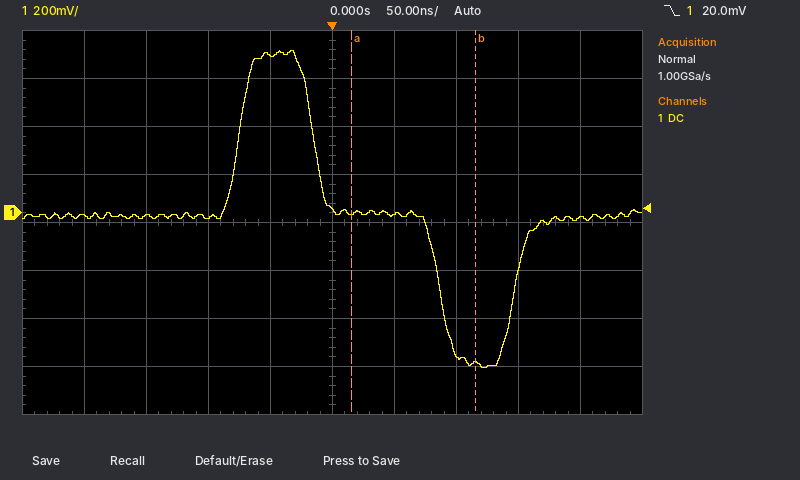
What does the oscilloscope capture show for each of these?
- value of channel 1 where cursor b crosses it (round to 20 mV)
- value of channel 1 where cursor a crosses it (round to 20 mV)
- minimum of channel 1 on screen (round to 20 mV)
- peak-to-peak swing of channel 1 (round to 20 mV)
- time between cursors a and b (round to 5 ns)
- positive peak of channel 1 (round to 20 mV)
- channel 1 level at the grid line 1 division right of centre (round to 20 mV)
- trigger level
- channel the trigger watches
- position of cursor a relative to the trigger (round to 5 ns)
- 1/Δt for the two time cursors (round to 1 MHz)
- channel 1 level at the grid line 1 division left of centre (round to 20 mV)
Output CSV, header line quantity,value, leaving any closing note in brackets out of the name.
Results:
quantity,value
value of channel 1 where cursor b crosses it,-620 mV
value of channel 1 where cursor a crosses it,0 mV
minimum of channel 1 on screen,-640 mV
peak-to-peak swing of channel 1,1.32 V
time between cursors a and b,100 ns
positive peak of channel 1,680 mV
channel 1 level at the grid line 1 division right of centre,0 mV
trigger level,20.0 mV
channel the trigger watches,channel 1
position of cursor a relative to the trigger,+15 ns
1/Δt for the two time cursors,10 MHz
channel 1 level at the grid line 1 division left of centre,660 mV
